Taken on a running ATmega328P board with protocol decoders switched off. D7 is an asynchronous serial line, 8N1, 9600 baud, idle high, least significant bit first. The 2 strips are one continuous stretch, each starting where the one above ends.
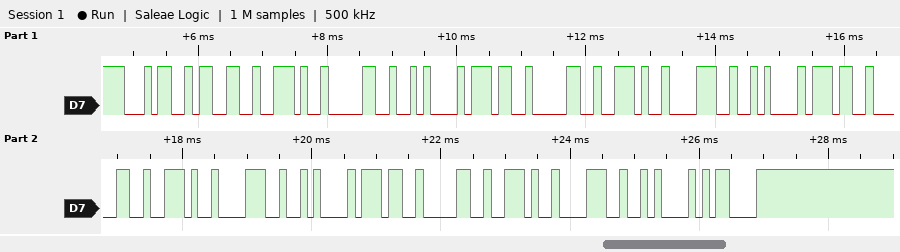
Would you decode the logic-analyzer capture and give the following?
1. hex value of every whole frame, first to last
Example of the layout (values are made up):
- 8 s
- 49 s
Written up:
- 0x34 0x33 0x2E 0x30 0x0A 0x37 0x30 0x2E 0x38 0x0A 0x37 0x30 0x2E 0x38 0x0A 0x37 0x30 0x2E 0x38 0x0A 0x0D
